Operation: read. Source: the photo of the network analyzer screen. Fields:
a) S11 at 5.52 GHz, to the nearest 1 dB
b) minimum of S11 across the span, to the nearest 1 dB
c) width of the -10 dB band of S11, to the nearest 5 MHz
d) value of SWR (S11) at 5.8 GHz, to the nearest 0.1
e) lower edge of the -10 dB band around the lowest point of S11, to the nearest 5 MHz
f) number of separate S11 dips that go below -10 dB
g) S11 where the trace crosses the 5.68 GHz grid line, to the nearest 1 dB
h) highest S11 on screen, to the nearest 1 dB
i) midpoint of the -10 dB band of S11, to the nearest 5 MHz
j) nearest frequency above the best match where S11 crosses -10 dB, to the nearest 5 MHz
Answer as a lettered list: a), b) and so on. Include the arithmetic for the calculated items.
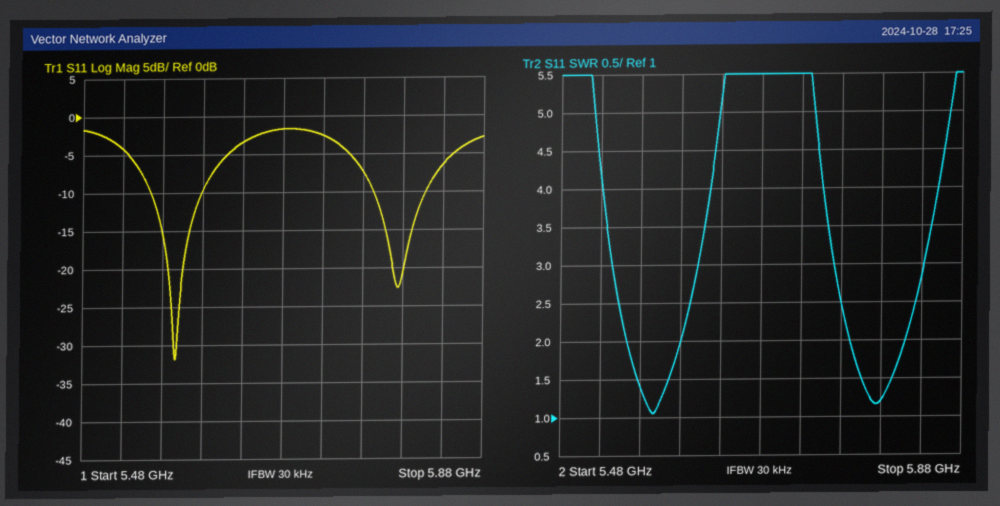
a) -4 dB
b) -32 dB
c) 5.600 GHz − 5.550 GHz = 50 MHz
d) 1.2
e) 5.550 GHz
f) 2
g) -2 dB
h) -2 dB
i) 5.575 GHz
j) 5.600 GHz
